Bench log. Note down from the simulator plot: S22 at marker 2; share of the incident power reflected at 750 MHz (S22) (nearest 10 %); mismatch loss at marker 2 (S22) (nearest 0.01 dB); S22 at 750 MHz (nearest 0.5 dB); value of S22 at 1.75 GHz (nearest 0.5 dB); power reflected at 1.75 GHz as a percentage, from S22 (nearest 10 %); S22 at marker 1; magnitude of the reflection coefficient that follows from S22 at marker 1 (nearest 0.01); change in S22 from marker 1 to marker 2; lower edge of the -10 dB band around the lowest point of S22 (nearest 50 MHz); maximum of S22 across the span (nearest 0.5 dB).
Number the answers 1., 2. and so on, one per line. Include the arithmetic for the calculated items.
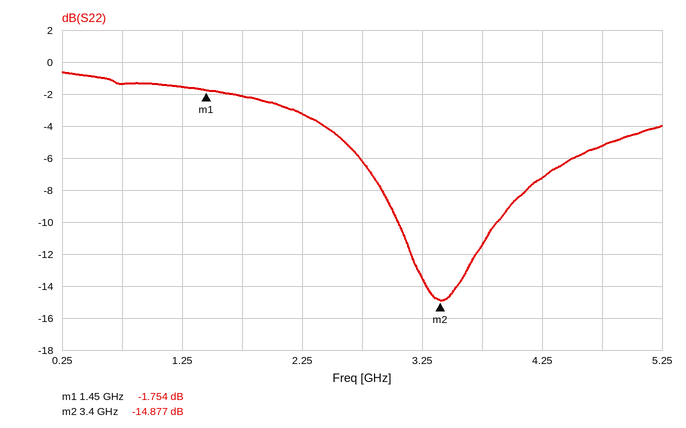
1. -14.877 dB
2. 10^(-1.5/10) ≈ 70.8 %, so 70 % to the nearest 10 %
3. −10 log10(1 − 10^(-14.877/10)) ≈ 0.14 dB
4. -1.5 dB
5. -2.0 dB
6. 10^(-2/10) ≈ 63.1 %, so 60 % to the nearest 10 %
7. -1.754 dB
8. 10^(-1.754/20) ≈ 0.82
9. -14.877 − (-1.754) = -13.123 dB
10. 3.05 GHz
11. -0.5 dB
